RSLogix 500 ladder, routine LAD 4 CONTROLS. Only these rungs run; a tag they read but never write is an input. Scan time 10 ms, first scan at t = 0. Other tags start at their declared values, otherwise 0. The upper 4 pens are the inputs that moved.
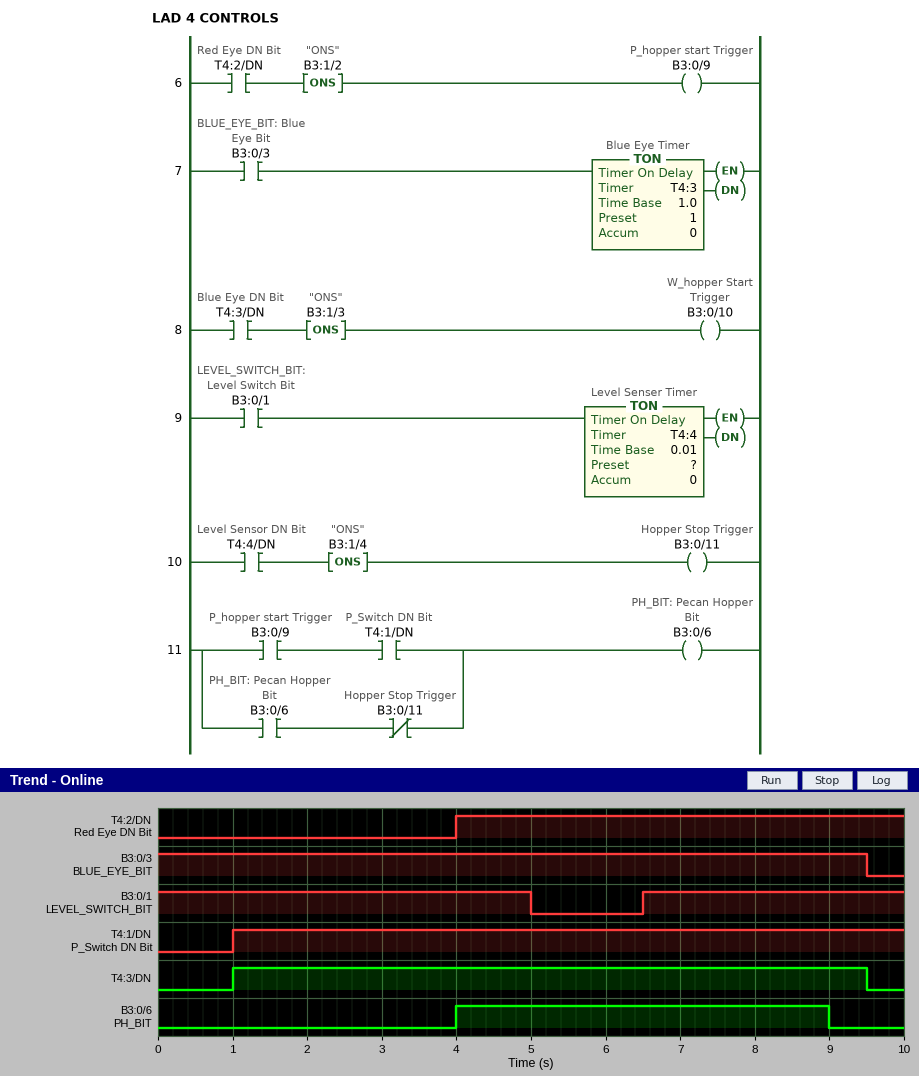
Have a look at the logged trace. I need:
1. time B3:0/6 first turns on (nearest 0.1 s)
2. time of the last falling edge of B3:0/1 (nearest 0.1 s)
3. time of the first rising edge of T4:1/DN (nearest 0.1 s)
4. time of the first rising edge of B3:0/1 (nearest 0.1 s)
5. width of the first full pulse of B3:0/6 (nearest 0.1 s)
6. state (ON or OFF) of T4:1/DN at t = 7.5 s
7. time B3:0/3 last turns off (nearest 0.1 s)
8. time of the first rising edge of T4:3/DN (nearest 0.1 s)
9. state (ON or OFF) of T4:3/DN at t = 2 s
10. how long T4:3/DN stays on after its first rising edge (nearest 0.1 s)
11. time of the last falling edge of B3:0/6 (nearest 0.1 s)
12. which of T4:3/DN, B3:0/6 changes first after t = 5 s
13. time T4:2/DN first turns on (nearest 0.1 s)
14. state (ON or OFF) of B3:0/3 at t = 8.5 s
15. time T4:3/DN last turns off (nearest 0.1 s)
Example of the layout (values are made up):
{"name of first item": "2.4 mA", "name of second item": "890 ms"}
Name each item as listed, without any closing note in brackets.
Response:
{"time B3:0/6 first turns on": "4.0 s", "time of the last falling edge of B3:0/1": "5.0 s", "time of the first rising edge of T4:1/DN": "1.0 s", "time of the first rising edge of B3:0/1": "6.5 s", "width of the first full pulse of B3:0/6": "5.0 s", "state (ON or OFF) of T4:1/DN at t = 7.5 s": "ON", "time B3:0/3 last turns off": "9.5 s", "time of the first rising edge of T4:3/DN": "1.0 s", "state (ON or OFF) of T4:3/DN at t = 2 s": "ON", "how long T4:3/DN stays on after its first rising edge": "8.5 s", "time of the last falling edge of B3:0/6": "9.0 s", "which of T4:3/DN, B3:0/6 changes first after t = 5 s": "B3:0/6", "time T4:2/DN first turns on": "4.0 s", "state (ON or OFF) of B3:0/3 at t = 8.5 s": "ON", "time T4:3/DN last turns off": "9.5 s"}
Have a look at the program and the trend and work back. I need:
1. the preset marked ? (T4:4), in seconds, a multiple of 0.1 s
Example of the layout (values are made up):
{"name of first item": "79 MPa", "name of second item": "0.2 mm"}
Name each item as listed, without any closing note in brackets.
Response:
{"the preset marked ? (T4:4), in seconds, a multiple of 0.1 s": "2.5 s"}
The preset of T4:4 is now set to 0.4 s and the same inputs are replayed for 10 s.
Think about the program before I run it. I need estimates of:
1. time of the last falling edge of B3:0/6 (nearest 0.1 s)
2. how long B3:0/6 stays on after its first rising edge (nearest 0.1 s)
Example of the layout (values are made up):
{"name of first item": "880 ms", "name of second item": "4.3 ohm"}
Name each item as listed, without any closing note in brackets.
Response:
{"time of the last falling edge of B3:0/6": "6.9 s", "how long B3:0/6 stays on after its first rising edge": "2.9 s"}
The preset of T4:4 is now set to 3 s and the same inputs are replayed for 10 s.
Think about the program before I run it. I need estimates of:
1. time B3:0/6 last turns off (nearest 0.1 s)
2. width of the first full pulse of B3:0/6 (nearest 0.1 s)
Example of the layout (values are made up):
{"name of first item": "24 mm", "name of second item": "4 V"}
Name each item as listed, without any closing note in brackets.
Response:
{"time B3:0/6 last turns off": "9.5 s", "width of the first full pulse of B3:0/6": "5.5 s"}
